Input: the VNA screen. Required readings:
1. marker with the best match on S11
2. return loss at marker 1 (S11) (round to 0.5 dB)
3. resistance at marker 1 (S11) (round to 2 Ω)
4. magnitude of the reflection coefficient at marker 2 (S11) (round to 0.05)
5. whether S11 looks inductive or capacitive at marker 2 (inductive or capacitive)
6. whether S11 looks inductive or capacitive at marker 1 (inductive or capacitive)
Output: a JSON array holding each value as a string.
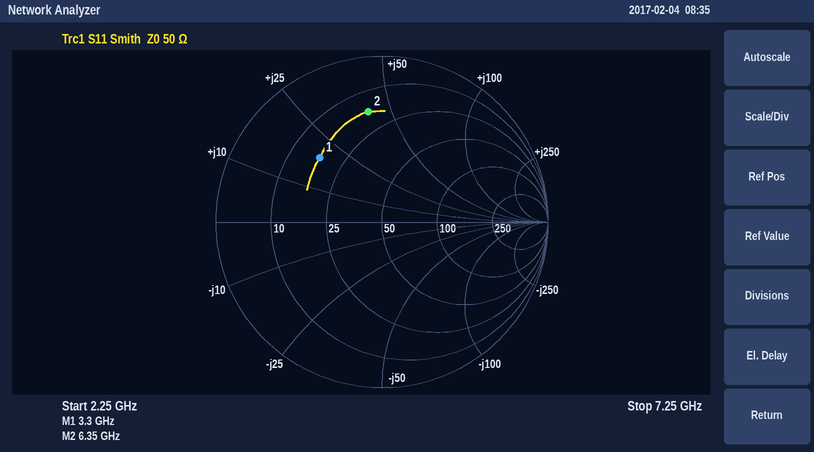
["marker 1", "5.5 dB", "18 Ω", "0.65", "inductive", "inductive"]
